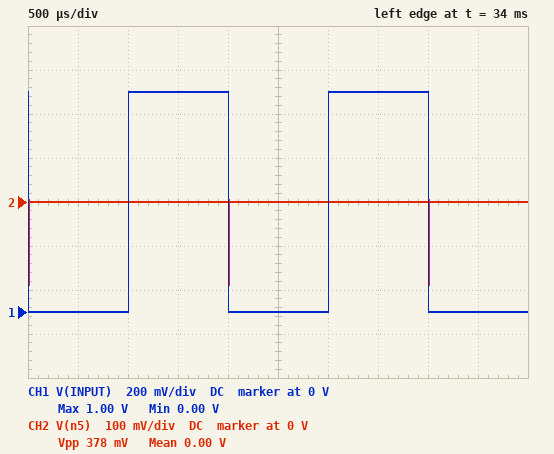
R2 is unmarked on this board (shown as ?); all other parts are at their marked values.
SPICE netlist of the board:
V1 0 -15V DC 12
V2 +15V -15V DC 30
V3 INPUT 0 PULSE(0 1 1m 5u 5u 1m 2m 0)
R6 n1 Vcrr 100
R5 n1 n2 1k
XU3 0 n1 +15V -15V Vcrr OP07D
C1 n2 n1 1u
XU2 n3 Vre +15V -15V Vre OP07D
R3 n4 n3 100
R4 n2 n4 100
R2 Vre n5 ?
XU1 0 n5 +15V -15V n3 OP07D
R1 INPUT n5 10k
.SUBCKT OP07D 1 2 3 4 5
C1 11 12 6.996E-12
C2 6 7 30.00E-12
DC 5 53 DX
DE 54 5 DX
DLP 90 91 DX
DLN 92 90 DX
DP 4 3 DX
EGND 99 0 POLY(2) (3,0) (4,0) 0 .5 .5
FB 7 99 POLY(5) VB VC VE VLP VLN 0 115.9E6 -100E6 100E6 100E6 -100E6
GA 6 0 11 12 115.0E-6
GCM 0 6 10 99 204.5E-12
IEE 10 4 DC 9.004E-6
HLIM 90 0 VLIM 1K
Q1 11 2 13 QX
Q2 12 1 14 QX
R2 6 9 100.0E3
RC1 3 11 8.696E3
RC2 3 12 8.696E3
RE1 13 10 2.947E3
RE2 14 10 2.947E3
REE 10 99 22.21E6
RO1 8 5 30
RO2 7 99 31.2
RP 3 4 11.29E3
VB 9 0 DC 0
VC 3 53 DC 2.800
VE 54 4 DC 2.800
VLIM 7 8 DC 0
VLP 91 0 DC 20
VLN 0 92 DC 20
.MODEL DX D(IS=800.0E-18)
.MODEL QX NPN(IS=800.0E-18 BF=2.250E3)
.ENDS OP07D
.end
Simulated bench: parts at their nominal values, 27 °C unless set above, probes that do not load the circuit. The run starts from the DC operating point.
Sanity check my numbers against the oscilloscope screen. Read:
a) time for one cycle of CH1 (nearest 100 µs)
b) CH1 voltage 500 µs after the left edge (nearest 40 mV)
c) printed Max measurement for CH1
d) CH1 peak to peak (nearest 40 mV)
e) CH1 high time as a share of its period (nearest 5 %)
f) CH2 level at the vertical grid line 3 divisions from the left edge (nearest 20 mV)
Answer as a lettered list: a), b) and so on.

a) 2.0 ms
b) 0 V
c) 1.00 V
d) 1.00 V
e) 50 %
f) 0 V
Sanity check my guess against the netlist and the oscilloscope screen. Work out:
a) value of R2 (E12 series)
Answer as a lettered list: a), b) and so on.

a) 15 kΩ
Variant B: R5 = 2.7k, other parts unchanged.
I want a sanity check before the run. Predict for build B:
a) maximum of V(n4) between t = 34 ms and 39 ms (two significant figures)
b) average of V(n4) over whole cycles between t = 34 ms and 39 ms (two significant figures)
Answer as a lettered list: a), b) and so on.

a) -3.3 mV
b) -730 mV
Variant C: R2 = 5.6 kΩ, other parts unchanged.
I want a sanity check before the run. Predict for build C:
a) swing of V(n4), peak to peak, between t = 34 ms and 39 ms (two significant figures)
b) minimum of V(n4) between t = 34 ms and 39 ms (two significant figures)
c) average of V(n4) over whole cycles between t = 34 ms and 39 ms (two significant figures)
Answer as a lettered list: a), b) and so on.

a) 510 mV
b) -510 mV
c) -260 mV
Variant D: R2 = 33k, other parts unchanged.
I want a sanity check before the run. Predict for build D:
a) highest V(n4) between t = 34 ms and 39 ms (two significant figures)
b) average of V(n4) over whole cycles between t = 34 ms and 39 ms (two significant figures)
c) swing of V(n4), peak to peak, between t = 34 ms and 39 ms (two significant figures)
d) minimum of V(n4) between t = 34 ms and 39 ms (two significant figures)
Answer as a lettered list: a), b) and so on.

a) -3.5 mV
b) -1.5 V
c) 3.0 V
d) -3.0 V
